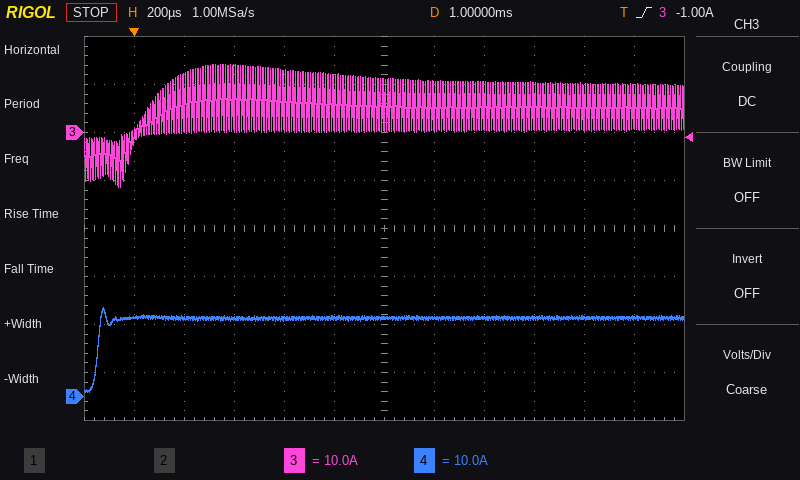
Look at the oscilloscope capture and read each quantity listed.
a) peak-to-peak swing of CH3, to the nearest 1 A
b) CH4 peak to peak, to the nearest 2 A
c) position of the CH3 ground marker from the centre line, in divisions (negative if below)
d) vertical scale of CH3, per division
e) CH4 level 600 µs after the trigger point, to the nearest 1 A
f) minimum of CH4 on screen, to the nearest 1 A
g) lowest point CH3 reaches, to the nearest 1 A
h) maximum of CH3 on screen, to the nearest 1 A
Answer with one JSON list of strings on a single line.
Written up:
["25 A", "18 A", "+2.0 div", "10 A", "16 A", "1 A", "-11 A", "14 A"]
